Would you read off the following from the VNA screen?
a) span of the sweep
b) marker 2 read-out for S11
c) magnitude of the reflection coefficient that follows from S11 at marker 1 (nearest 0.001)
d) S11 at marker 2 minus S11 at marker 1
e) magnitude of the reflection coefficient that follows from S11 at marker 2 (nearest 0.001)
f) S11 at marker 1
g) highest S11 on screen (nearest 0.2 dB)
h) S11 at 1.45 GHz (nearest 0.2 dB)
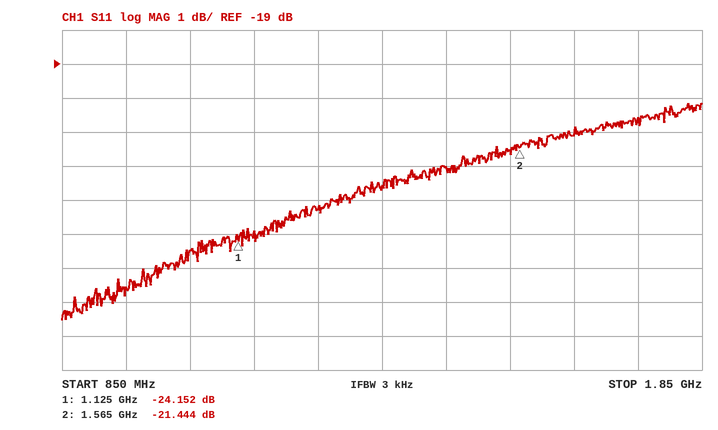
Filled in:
1 GHz
-21.444 dB
0.062
2.708 dB
0.085
-24.152 dB
-20.2 dB
-22.0 dB
